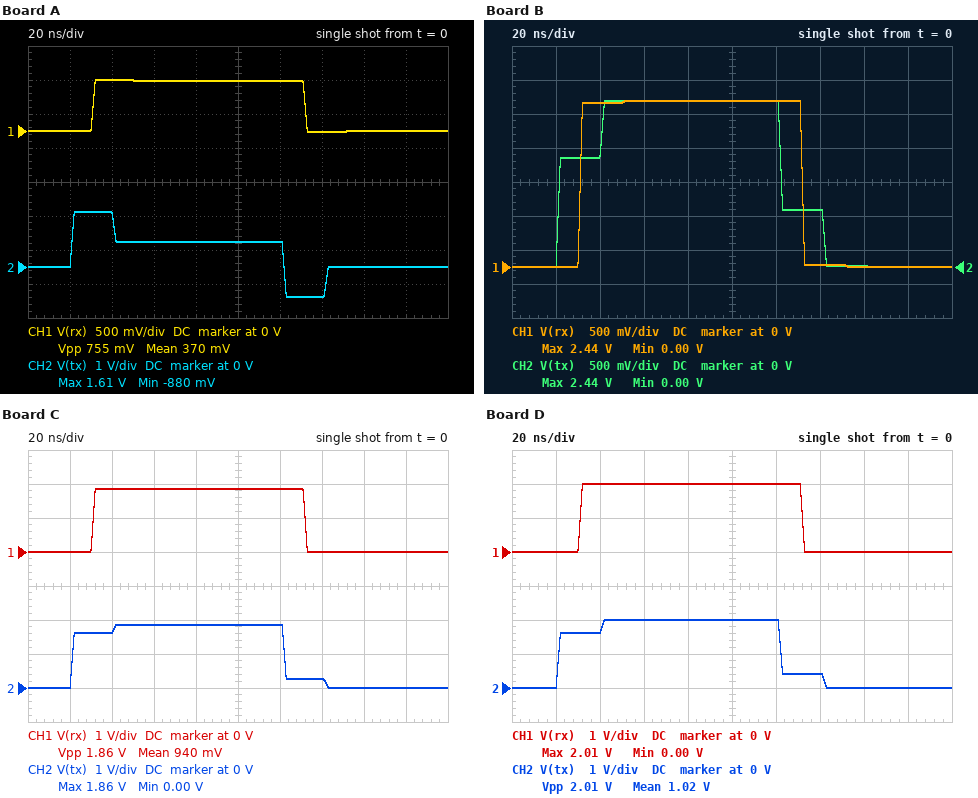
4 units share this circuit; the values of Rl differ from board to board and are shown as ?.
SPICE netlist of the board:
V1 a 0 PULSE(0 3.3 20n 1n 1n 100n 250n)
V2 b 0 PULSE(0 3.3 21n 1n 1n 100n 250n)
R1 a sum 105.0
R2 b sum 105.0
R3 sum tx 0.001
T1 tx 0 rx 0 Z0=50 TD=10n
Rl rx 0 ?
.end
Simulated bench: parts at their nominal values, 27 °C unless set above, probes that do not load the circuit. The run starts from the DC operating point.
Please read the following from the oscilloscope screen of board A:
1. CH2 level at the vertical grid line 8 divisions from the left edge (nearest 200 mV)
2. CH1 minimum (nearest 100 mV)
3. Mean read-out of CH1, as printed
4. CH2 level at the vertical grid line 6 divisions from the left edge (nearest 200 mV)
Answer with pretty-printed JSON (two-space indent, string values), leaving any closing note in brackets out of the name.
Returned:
{
  "CH2 level at the vertical grid line 8 divisions from the left edge": "0 V",
  "CH1 minimum": "0 V",
  "Mean read-out of CH1, as printed": "370 mV",
  "CH2 level at the vertical grid line 6 divisions from the left edge": "800 mV"
}
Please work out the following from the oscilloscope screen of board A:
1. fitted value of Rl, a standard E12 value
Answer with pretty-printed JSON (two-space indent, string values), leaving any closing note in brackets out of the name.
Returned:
{
  "fitted value of Rl, a standard E12 value": "15 Ω"
}
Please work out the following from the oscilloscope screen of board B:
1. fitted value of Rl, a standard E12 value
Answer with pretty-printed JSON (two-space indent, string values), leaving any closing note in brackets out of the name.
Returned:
{
  "fitted value of Rl, a standard E12 value": "150 Ω"
}
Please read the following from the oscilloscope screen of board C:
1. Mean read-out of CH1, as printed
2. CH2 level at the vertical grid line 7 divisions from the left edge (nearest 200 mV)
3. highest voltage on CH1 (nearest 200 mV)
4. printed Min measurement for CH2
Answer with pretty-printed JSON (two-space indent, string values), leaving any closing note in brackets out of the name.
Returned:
{
  "Mean read-out of CH1, as printed": "940 mV",
  "CH2 level at the vertical grid line 7 divisions from the left edge": "200 mV",
  "highest voltage on CH1": "1.8 V",
  "printed Min measurement for CH2": "0.00 V"
}
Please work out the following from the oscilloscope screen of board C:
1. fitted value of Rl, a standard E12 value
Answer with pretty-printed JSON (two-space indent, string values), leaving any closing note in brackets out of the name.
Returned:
{
  "fitted value of Rl, a standard E12 value": "68 Ω"
}
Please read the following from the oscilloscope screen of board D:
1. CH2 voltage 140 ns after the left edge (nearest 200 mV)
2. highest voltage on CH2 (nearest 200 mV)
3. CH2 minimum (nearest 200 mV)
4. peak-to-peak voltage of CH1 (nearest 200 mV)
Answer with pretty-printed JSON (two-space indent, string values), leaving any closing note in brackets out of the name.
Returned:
{
  "CH2 voltage 140 ns after the left edge": "400 mV",
  "highest voltage on CH2": "2.0 V",
  "CH2 minimum": "0 V",
  "peak-to-peak voltage of CH1": "2.0 V"
}
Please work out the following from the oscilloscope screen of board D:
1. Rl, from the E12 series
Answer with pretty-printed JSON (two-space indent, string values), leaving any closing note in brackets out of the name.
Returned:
{
  "Rl, from the E12 series": "82 Ω"
}
